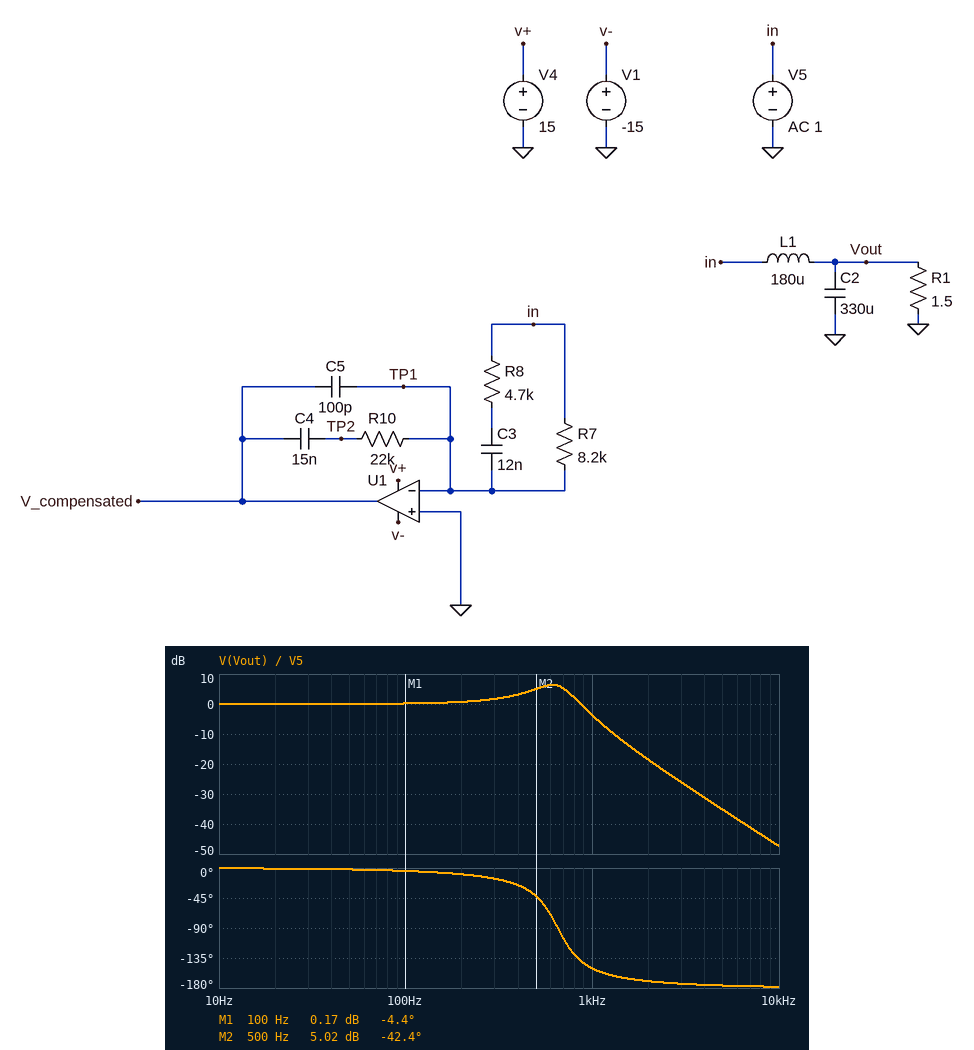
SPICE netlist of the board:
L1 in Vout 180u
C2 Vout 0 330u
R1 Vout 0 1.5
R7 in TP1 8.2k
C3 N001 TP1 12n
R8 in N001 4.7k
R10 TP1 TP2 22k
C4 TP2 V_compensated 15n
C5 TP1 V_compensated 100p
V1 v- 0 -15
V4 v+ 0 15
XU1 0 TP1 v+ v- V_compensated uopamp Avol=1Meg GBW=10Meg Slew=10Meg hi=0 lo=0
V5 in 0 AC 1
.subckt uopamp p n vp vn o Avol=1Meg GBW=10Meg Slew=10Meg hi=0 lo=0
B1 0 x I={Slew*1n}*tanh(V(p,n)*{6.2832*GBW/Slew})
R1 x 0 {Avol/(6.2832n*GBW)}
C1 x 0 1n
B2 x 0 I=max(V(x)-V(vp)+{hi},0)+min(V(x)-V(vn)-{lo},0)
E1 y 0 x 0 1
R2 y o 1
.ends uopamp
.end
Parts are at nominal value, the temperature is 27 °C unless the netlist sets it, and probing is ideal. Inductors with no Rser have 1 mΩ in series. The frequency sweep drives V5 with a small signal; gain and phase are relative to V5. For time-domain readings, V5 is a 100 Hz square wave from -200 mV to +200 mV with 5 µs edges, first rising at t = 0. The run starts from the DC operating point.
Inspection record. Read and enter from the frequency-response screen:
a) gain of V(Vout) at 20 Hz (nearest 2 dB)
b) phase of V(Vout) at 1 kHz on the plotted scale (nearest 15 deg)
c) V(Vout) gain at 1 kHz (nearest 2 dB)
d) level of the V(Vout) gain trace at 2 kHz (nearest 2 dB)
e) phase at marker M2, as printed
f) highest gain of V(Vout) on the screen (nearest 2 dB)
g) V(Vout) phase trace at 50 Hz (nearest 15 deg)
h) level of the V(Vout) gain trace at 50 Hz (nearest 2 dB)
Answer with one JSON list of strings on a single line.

["0 dB", "-150 deg", "-4 dB", "-18 dB", "-42.4 deg", "6 dB", "0 deg", "0 dB"]
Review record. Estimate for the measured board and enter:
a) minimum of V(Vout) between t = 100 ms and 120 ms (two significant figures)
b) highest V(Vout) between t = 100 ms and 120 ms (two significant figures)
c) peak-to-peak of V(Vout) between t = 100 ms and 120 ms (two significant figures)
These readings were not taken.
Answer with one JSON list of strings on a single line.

["-380 mV", "380 mV", "760 mV"]
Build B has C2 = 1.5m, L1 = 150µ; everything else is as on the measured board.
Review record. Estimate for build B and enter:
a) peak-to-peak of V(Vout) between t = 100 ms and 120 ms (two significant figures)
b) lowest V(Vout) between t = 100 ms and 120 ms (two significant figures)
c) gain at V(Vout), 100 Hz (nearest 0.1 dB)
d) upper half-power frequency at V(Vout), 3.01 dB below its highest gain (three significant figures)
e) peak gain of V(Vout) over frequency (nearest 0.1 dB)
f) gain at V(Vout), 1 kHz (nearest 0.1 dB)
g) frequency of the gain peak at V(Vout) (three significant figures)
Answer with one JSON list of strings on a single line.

["1.1 V", "-530 mV", "0.8 dB", "366 Hz", "13.4 dB", "-18.0 dB", "332 Hz"]
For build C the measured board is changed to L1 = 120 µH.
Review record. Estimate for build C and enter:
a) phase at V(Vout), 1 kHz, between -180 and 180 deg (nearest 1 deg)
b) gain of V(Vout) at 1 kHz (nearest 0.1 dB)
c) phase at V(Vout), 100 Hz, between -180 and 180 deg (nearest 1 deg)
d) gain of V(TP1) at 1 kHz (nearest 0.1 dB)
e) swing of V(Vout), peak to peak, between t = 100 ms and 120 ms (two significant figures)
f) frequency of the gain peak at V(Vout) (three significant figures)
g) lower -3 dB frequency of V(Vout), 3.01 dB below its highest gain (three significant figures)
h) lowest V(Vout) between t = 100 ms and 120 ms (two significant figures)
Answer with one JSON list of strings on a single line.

["-138 deg", "2.4 dB", "-3 deg", "-68.2 dB", "820 mV", "767 Hz", "579 Hz", "-410 mV"]
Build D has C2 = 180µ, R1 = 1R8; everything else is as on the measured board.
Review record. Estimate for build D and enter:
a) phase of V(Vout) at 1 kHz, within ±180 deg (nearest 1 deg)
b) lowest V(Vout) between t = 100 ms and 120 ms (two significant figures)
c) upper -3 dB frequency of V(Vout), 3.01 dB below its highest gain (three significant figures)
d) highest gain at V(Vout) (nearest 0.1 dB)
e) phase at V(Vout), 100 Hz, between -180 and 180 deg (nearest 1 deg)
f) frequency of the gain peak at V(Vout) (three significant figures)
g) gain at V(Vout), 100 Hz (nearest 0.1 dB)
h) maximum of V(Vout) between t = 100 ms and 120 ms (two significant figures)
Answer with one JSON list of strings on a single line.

["-114 deg", "-360 mV", "1.04 kHz", "5.4 dB", "-4 deg", "813 Hz", "0.1 dB", "360 mV"]
